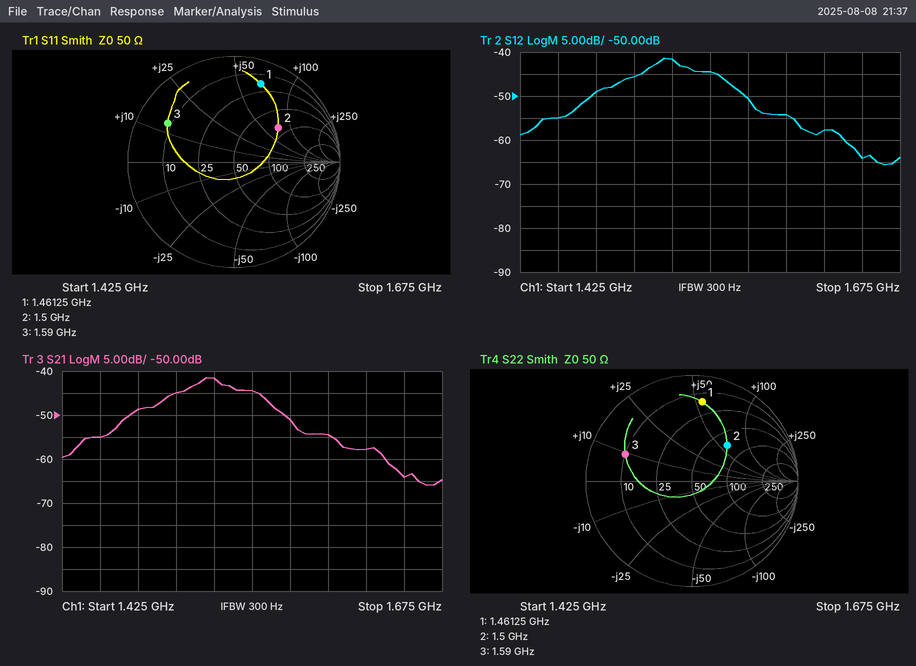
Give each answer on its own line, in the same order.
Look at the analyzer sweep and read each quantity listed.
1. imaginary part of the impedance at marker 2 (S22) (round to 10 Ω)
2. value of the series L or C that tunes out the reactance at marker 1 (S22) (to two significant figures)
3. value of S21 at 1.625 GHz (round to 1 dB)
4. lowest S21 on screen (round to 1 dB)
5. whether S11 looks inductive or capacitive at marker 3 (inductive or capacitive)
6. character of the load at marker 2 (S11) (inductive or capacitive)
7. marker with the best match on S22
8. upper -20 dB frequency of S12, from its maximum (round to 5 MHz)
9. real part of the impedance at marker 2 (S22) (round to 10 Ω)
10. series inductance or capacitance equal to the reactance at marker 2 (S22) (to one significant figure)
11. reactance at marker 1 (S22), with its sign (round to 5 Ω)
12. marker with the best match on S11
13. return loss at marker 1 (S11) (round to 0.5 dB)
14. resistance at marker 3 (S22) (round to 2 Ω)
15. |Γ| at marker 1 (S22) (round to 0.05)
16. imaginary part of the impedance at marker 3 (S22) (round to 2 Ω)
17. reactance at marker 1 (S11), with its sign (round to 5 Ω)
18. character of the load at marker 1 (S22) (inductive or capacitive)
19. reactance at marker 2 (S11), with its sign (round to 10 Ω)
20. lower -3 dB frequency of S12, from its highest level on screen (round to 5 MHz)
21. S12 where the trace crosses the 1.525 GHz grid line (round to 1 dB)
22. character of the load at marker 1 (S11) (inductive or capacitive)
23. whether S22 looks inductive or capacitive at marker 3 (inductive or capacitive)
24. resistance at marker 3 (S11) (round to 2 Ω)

+60 Ω
2.0 pF
-58 dB
-66 dB
inductive
inductive
marker 2
1.645 GHz
70 Ω
6 nH
+55 Ω
marker 2
2.0 dB
10 Ω
0.75
+10 Ω
+65 Ω
inductive
+70 Ω
1.505 GHz
-42 dB
inductive
inductive
8 Ω
